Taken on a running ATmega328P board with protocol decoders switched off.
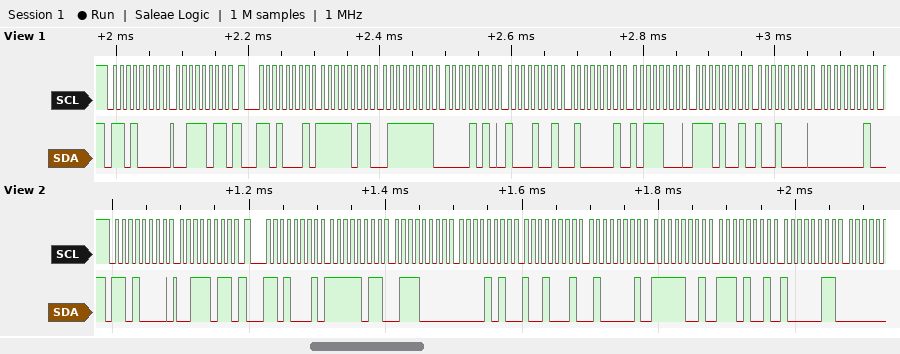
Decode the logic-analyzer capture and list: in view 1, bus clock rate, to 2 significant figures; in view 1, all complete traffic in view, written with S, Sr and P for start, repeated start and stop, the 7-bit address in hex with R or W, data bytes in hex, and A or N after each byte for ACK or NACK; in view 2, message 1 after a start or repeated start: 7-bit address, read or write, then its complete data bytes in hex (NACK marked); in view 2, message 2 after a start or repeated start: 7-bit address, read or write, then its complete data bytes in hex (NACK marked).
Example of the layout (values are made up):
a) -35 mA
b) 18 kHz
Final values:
a) 100 kHz
b) S 68W A 3B A Sr 68R A FB A 7F A 0A A 89 A 41 A B8 A E9 A 90 A 01 A
c) 0x68 write: 3B
d) 0x68 read: FB 70 0A 91 41 F9 E9 83
